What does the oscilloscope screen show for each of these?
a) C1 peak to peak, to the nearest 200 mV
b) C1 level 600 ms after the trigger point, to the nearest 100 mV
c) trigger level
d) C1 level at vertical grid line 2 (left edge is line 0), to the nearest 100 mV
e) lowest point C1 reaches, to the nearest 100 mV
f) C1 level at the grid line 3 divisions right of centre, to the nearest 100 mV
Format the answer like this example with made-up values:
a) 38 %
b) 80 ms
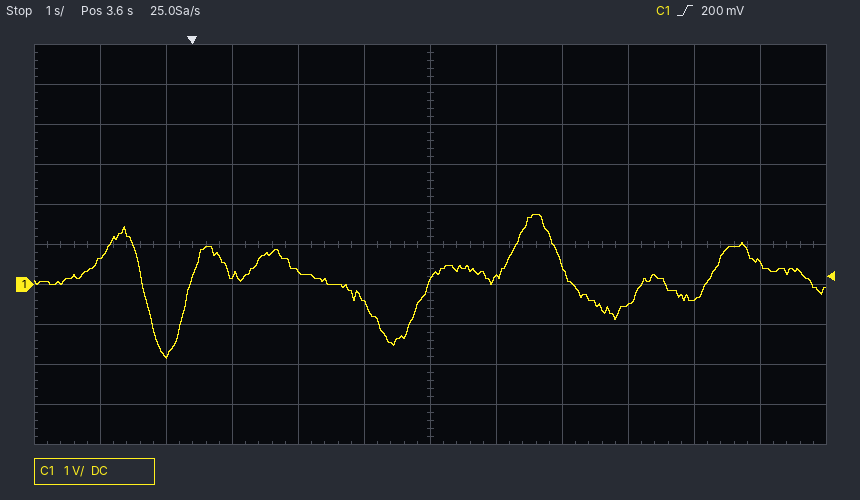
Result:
a) 3.6 V
b) 200 mV
c) 200 mV
d) -1.8 V
e) -1.8 V
f) -500 mV
